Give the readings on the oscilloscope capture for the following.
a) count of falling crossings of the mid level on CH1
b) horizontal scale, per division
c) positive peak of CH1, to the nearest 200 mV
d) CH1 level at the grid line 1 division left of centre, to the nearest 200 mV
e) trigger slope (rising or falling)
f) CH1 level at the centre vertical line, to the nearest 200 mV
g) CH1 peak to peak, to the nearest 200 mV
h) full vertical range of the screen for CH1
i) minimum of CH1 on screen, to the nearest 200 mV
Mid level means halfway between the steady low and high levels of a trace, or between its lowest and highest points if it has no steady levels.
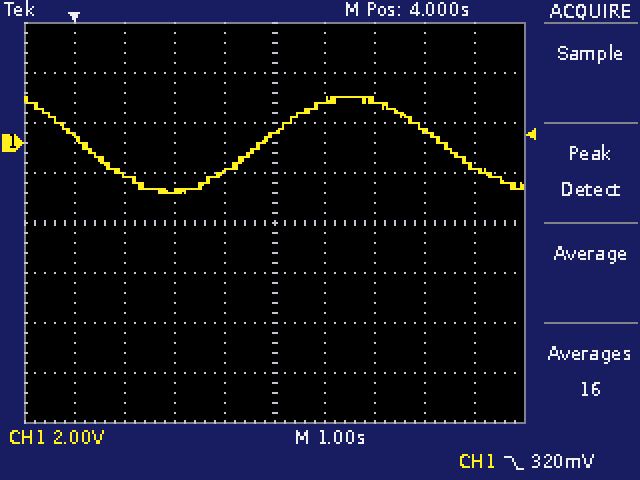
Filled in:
2
1 s
1.8 V
-1.2 V
falling
400 mV
3.8 V
16 V
-2.0 V
